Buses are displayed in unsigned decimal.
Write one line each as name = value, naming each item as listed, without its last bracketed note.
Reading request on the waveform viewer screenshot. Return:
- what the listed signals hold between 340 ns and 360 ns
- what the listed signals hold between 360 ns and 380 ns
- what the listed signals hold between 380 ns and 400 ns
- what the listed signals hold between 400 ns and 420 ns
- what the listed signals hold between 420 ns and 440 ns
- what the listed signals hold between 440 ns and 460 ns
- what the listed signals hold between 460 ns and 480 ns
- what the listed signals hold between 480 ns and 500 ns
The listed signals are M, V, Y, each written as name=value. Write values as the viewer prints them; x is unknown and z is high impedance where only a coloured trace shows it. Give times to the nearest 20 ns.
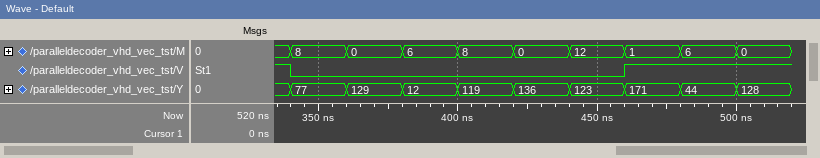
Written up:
what the listed signals hold between 340 ns and 360 ns = M=8, V=0, Y=77
what the listed signals hold between 360 ns and 380 ns = M=0, V=0, Y=129
what the listed signals hold between 380 ns and 400 ns = M=6, V=0, Y=12
what the listed signals hold between 400 ns and 420 ns = M=8, V=0, Y=119
what the listed signals hold between 420 ns and 440 ns = M=0, V=0, Y=136
what the listed signals hold between 440 ns and 460 ns = M=12, V=0, Y=123
what the listed signals hold between 460 ns and 480 ns = M=1, V=1, Y=171
what the listed signals hold between 480 ns and 500 ns = M=6, V=1, Y=44
